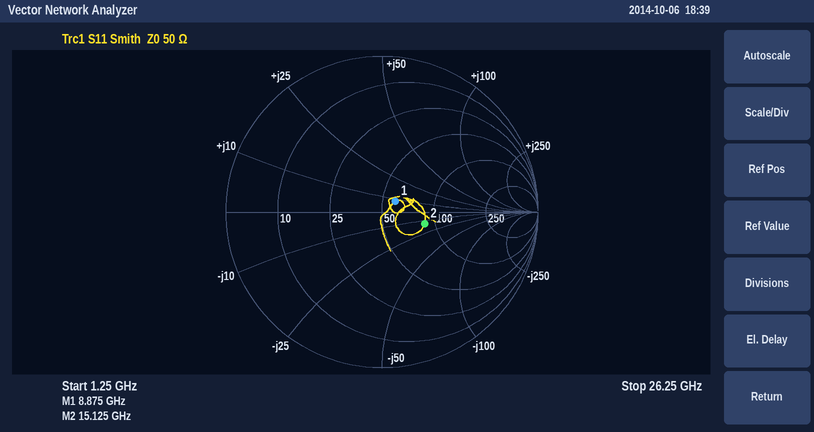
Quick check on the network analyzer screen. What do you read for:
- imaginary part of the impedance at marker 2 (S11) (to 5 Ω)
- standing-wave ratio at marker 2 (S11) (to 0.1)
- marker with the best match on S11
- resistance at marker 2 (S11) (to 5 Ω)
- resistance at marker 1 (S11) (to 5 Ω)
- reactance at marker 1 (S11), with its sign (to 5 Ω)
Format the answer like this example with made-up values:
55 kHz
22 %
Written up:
-15 Ω
1.8
marker 1
85 Ω
60 Ω
+10 Ω
